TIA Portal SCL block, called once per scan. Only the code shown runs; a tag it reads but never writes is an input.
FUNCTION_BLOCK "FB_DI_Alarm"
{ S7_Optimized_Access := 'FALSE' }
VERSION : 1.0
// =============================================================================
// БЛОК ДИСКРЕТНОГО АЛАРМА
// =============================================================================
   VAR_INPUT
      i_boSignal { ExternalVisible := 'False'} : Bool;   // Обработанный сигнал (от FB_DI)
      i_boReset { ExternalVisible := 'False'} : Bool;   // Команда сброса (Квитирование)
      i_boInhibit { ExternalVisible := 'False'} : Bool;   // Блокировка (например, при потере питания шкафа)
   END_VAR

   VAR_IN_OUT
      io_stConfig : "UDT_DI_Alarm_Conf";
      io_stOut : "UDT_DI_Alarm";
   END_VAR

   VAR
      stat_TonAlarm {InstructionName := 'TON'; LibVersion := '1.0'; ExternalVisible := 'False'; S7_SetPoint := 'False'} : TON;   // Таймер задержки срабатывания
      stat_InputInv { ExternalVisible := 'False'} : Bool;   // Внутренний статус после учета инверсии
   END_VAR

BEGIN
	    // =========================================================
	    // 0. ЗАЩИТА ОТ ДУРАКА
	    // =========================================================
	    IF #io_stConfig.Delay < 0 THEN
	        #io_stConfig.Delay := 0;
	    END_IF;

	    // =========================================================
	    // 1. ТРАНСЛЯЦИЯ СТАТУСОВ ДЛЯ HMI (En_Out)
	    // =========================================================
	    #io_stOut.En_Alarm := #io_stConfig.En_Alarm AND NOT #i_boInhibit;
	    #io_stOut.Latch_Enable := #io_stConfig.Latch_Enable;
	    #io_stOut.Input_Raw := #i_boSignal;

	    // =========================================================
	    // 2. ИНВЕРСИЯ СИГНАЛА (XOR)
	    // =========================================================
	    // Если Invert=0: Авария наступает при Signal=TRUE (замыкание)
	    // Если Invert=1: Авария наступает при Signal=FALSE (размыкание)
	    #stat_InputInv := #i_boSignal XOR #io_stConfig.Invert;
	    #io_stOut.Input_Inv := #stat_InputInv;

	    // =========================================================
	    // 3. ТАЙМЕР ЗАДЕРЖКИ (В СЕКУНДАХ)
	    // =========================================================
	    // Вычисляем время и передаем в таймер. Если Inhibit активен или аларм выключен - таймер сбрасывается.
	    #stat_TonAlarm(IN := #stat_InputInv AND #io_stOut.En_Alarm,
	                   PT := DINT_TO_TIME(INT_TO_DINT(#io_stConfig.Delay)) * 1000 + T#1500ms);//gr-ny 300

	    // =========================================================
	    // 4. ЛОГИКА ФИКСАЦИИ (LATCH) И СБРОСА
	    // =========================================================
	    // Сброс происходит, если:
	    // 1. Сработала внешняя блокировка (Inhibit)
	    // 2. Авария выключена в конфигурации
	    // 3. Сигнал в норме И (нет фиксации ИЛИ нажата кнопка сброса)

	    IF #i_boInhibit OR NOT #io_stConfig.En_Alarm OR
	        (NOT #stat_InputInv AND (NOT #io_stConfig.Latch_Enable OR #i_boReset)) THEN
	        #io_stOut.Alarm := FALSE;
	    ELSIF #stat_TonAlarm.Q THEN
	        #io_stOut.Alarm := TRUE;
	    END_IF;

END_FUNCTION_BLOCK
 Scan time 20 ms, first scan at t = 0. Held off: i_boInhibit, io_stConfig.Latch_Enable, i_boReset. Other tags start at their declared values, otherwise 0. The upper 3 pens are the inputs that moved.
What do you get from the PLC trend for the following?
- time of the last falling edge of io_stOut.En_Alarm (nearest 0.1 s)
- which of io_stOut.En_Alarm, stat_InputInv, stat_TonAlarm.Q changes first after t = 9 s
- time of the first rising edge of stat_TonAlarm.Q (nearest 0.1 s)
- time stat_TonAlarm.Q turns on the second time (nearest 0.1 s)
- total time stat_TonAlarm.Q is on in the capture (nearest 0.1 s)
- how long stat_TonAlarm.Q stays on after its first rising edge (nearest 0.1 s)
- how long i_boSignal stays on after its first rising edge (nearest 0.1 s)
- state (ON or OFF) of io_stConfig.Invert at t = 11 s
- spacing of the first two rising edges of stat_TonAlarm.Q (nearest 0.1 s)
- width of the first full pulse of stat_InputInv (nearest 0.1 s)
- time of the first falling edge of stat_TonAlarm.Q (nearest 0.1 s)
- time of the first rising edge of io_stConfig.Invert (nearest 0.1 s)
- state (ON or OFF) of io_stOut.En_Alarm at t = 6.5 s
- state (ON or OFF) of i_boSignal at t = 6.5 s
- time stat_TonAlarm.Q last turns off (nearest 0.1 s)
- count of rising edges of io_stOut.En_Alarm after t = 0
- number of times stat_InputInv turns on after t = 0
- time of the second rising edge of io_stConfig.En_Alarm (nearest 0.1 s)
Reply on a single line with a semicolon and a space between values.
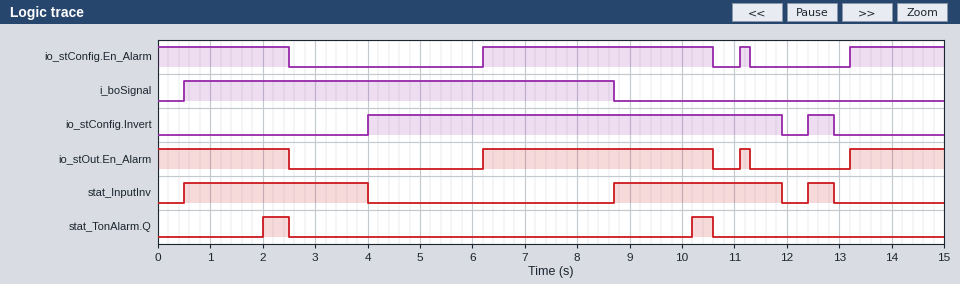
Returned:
11.3 s; stat_TonAlarm.Q; 2.0 s; 10.2 s; 0.9 s; 0.5 s; 8.2 s; ON; 8.2 s; 3.5 s; 2.5 s; 4.0 s; ON; ON; 10.6 s; 3; 3; 11.1 s
